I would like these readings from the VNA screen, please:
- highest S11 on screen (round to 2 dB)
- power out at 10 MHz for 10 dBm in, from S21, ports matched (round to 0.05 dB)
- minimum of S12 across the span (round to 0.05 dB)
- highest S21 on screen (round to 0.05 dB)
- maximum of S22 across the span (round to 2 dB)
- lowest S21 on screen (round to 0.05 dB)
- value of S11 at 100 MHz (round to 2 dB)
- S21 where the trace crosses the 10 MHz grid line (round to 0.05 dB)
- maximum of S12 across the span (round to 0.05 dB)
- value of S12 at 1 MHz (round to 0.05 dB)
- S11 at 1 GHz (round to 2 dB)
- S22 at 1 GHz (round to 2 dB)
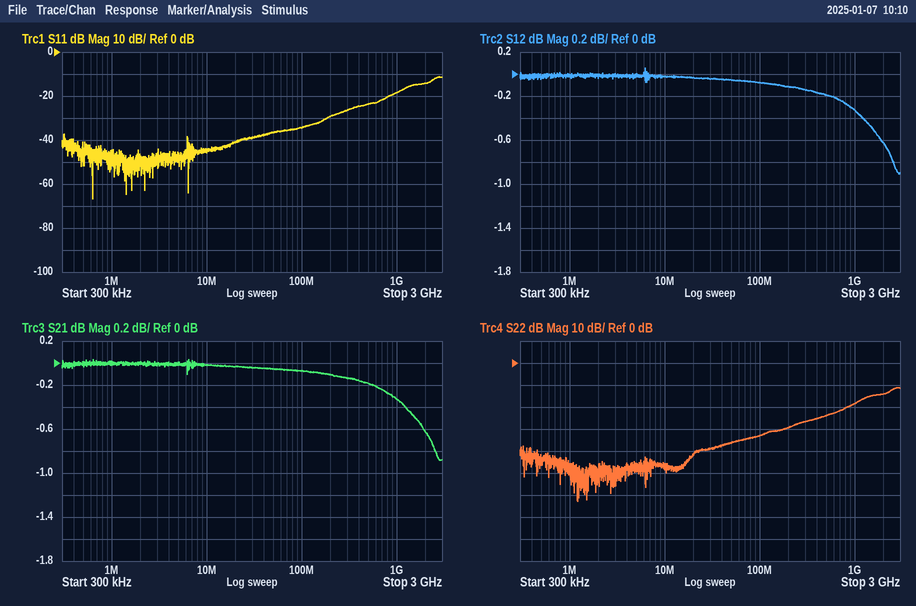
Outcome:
-12 dB
10.00 dBm
-0.90 dB
0.05 dB
-12 dB
-0.90 dB
-34 dB
0.00 dB
0.05 dB
0.00 dB
-18 dB
-18 dB
